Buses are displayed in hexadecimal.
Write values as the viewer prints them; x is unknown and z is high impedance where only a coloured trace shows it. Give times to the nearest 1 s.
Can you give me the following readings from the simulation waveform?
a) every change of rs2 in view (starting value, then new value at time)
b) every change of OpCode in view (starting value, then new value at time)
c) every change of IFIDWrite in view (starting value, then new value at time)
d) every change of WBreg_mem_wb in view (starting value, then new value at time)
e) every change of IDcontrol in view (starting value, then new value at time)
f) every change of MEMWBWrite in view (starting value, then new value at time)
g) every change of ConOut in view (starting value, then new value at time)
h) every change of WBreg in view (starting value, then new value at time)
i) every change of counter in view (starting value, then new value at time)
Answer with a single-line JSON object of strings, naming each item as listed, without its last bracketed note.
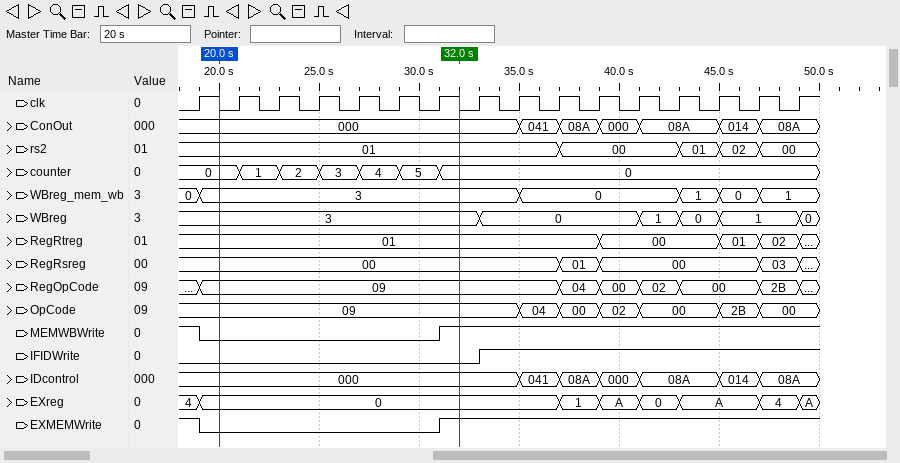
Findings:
{"every change of rs2 in view": "01, 00 at 37 s, 01 at 43 s, 02 at 45 s, 00 at 47 s", "every change of OpCode in view": "09, 04 at 35 s, 00 at 37 s, 02 at 39 s, 00 at 41 s, 2B at 45 s, 00 at 47 s", "every change of IFIDWrite in view": "0, 1 at 33 s", "every change of WBreg_mem_wb in view": "0, 3 at 19 s, 0 at 35 s, 1 at 43 s, 0 at 45 s, 1 at 47 s", "every change of IDcontrol in view": "000, 041 at 35 s, 08A at 37 s, 000 at 39 s, 08A at 41 s, 014 at 45 s, 08A at 47 s", "every change of MEMWBWrite in view": "1, 0 at 19 s, 1 at 31 s", "every change of ConOut in view": "000, 041 at 35 s, 08A at 37 s, 000 at 39 s, 08A at 41 s, 014 at 45 s, 08A at 47 s", "every change of WBreg in view": "3, 0 at 33 s, 1 at 41 s, 0 at 43 s, 1 at 45 s, 0 at 49 s", "every change of counter in view": "0, 1 at 21 s, 2 at 23 s, 3 at 25 s, 4 at 27 s, 5 at 29 s, 0 at 31 s"}
